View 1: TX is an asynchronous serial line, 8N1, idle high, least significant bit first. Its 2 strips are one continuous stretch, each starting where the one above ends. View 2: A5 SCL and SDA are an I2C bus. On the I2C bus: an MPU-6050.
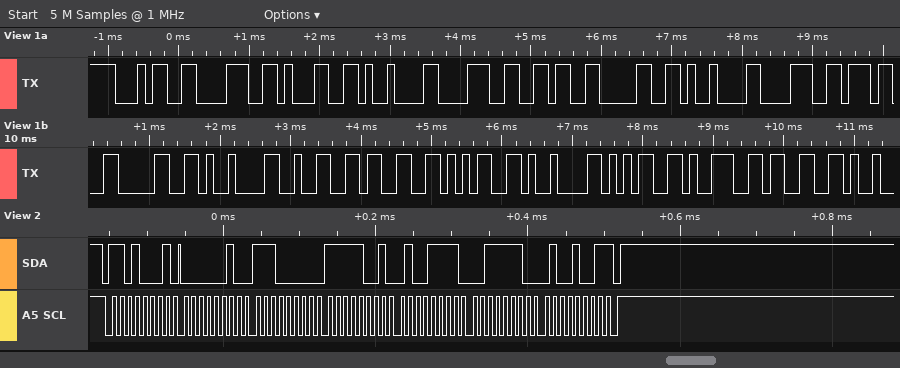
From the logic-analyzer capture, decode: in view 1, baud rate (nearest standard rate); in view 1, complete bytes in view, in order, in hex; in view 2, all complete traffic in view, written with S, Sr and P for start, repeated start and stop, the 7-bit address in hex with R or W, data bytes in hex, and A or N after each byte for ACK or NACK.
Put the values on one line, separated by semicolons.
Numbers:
9600 baud; 0x34 0x38 0x31 0x09 0x38 0x36 0x30 0x09 0x38 0x37 0x30 0x09 0x32 0x33 0x35 0x09 0x35 0x39 0x33; S 68R A 02 A E0 A F9 A 4F A 3E A 49 N P
